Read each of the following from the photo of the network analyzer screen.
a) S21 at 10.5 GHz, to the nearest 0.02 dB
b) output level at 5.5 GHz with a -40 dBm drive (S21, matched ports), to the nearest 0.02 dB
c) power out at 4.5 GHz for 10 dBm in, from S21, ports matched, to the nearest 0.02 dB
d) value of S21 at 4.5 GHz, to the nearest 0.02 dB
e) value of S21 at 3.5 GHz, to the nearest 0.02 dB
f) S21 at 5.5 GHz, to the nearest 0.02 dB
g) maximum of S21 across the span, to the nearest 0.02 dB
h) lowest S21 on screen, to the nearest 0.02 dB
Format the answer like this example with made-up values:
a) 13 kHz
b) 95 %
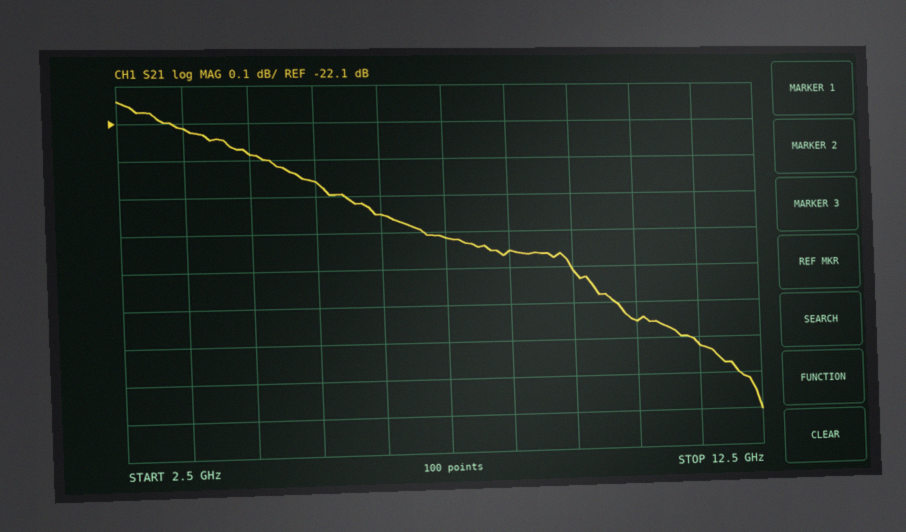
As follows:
a) -22.66 dB
b) -62.26 dBm
c) -12.18 dBm
d) -22.18 dB
e) -22.12 dB
f) -22.26 dB
g) -22.04 dB
h) -22.90 dB
